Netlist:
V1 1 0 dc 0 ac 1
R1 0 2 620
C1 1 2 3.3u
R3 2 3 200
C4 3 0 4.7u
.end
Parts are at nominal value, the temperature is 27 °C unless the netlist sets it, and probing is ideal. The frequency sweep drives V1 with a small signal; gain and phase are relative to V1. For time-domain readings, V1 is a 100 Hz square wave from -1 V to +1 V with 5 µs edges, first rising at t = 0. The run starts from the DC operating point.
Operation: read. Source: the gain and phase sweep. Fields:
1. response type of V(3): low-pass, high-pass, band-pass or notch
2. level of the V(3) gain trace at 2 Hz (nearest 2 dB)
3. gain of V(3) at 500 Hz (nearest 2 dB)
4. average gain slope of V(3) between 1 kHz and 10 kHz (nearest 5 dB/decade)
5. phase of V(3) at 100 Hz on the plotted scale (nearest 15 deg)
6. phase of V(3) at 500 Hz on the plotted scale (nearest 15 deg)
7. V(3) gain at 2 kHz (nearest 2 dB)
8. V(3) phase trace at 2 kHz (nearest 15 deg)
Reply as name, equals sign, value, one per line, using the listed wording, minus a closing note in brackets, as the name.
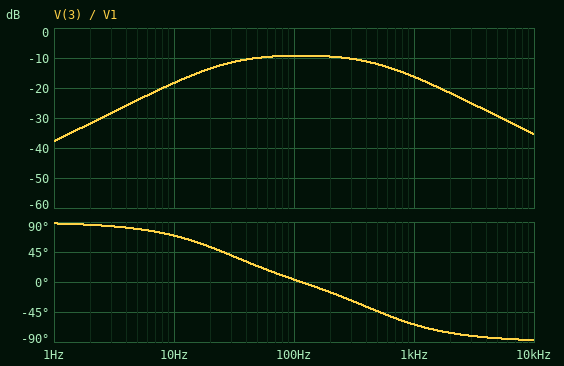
response type of V(3): low-pass, high-pass, band-pass or notch = band-pass
level of the V(3) gain trace at 2 Hz = -32 dB
gain of V(3) at 500 Hz = -12 dB
average gain slope of V(3) between 1 kHz and 10 kHz = -20 dB/decade
phase of V(3) at 100 Hz on the plotted scale = 0 deg
phase of V(3) at 500 Hz on the plotted scale = -45 deg
V(3) gain at 2 kHz = -22 dB
V(3) phase trace at 2 kHz = -75 deg
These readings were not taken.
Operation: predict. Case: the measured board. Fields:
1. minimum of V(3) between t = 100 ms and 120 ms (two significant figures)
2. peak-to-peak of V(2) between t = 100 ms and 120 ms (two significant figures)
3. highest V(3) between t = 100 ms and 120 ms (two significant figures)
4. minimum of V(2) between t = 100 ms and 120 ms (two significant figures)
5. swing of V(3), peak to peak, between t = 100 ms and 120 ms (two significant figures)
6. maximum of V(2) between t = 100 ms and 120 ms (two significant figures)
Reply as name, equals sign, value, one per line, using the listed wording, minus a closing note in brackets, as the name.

minimum of V(3) between t = 100 ms and 120 ms = -430 mV
peak-to-peak of V(2) between t = 100 ms and 120 ms = 3.6 V
highest V(3) between t = 100 ms and 120 ms = 430 mV
minimum of V(2) between t = 100 ms and 120 ms = -1.8 V
swing of V(3), peak to peak, between t = 100 ms and 120 ms = 850 mV
maximum of V(2) between t = 100 ms and 120 ms = 1.8 V
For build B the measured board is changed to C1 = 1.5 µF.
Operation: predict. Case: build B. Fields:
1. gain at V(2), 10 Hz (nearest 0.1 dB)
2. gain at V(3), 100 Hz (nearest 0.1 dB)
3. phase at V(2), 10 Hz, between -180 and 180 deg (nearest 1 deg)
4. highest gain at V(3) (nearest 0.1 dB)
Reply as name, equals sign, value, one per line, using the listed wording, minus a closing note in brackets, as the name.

gain at V(2), 10 Hz = -25.0 dB
gain at V(3), 100 Hz = -14.4 dB
phase at V(2), 10 Hz, between -180 and 180 deg = 77 deg
highest gain at V(3) = -14.2 dB
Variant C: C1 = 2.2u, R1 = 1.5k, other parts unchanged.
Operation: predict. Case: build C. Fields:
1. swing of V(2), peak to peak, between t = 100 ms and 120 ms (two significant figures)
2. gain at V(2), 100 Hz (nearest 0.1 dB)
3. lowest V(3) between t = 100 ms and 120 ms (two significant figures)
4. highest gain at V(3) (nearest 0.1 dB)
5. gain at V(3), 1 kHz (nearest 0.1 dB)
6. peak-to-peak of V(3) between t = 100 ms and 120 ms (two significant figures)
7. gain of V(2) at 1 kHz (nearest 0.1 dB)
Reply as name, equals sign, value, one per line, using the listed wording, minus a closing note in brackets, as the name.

swing of V(2), peak to peak, between t = 100 ms and 120 ms = 3.5 V
gain at V(2), 100 Hz = -9.4 dB
lowest V(3) between t = 100 ms and 120 ms = -330 mV
highest gain at V(3) = -10.7 dB
gain at V(3), 1 kHz = -16.6 dB
peak-to-peak of V(3) between t = 100 ms and 120 ms = 660 mV
gain of V(2) at 1 kHz = -1.1 dB
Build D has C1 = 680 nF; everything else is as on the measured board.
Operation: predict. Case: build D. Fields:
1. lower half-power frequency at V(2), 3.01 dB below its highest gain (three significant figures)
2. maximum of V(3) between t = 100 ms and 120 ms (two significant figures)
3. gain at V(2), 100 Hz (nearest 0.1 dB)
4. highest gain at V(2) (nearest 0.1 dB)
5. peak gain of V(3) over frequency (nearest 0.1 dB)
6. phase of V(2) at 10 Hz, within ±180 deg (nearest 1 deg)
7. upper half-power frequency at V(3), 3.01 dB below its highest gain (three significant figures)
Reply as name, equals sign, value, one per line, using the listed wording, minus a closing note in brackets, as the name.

lower half-power frequency at V(2), 3.01 dB below its highest gain = 1.66 kHz
maximum of V(3) between t = 100 ms and 120 ms = 140 mV
gain at V(2), 100 Hz = -19.2 dB
highest gain at V(2) = 0 dB
peak gain of V(3) over frequency = -20.1 dB
phase of V(2) at 10 Hz, within ±180 deg = 78 deg
upper half-power frequency at V(3), 3.01 dB below its highest gain = 1.75 kHz
